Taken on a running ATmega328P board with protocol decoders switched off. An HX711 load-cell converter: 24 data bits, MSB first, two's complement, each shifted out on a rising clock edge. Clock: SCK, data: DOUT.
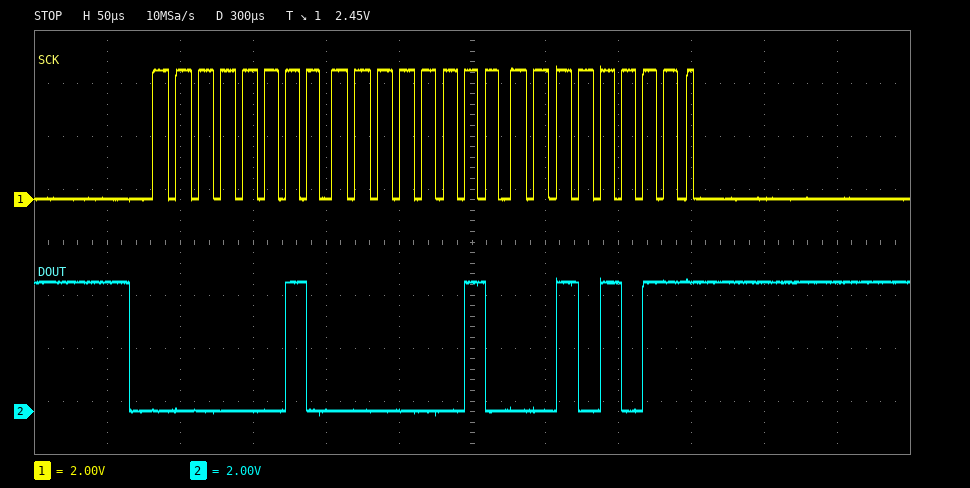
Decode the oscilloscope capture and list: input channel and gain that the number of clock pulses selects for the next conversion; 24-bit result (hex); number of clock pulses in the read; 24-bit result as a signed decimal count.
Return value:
channel A, gain 128
0x02022B
25
131627
